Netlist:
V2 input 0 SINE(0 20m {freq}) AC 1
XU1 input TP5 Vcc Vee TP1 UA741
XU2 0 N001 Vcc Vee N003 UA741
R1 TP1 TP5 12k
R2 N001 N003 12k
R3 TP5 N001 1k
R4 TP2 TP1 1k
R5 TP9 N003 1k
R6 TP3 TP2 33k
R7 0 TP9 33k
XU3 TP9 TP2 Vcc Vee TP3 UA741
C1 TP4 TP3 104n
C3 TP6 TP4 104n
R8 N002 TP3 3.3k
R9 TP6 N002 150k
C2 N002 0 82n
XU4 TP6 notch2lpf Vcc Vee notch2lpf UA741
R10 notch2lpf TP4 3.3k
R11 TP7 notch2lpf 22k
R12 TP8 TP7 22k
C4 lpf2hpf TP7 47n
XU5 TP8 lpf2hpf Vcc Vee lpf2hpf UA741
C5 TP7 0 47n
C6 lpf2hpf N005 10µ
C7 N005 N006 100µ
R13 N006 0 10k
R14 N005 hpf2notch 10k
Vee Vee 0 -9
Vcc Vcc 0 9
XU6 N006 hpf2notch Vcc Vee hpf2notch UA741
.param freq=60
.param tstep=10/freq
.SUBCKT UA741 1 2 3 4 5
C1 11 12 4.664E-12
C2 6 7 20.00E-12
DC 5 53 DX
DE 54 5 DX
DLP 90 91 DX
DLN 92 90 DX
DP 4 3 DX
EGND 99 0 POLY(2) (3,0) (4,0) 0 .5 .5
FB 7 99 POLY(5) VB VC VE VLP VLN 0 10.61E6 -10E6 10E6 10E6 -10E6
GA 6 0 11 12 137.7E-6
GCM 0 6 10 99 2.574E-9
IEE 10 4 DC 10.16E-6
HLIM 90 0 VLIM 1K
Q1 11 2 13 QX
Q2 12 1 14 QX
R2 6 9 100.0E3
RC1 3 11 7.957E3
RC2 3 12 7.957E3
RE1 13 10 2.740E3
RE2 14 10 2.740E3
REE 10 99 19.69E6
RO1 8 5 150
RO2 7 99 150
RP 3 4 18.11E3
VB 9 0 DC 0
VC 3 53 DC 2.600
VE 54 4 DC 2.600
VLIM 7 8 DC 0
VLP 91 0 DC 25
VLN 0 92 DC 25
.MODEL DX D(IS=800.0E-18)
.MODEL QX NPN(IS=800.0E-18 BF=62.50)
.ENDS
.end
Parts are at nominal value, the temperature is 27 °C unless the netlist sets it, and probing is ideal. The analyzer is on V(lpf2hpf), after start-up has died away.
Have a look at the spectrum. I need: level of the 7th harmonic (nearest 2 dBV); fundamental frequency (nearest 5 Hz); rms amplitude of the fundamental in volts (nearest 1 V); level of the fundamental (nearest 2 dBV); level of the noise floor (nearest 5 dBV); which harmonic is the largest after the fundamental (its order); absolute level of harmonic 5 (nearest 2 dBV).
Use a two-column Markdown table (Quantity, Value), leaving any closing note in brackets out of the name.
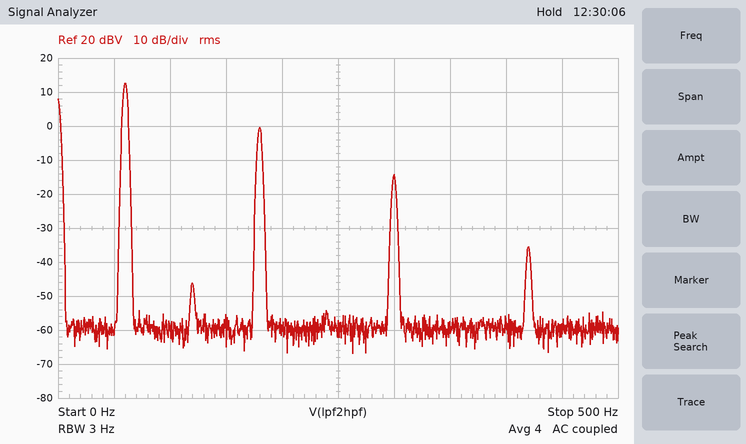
| Quantity | Value |
|---|---|
| level of the 7th harmonic | -36 dBV |
| fundamental frequency | 60 Hz |
| rms amplitude of the fundamental in volts | 4 V |
| level of the fundamental | 12 dBV |
| level of the noise floor | -60 dBV |
| which harmonic is the largest after the fundamental | 3 |
| absolute level of harmonic 5 | -14 dBV |
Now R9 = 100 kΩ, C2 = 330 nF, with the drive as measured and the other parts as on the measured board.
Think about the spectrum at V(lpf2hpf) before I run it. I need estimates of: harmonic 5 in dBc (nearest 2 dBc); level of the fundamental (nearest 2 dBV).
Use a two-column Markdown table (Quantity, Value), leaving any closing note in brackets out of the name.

| Quantity | Value |
|---|---|
| harmonic 5 in dBc | -30 dBc |
| level of the fundamental | 12 dBV |
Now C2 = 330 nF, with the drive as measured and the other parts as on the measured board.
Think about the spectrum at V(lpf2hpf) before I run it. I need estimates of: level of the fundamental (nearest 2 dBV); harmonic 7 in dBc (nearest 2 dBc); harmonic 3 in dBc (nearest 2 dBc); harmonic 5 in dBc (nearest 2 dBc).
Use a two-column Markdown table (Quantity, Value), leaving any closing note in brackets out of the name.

| Quantity | Value |
|---|---|
| level of the fundamental | 10 dBV |
| harmonic 7 in dBc | -50 dBc |
| harmonic 3 in dBc | -10 dBc |
| harmonic 5 in dBc | -24 dBc |
